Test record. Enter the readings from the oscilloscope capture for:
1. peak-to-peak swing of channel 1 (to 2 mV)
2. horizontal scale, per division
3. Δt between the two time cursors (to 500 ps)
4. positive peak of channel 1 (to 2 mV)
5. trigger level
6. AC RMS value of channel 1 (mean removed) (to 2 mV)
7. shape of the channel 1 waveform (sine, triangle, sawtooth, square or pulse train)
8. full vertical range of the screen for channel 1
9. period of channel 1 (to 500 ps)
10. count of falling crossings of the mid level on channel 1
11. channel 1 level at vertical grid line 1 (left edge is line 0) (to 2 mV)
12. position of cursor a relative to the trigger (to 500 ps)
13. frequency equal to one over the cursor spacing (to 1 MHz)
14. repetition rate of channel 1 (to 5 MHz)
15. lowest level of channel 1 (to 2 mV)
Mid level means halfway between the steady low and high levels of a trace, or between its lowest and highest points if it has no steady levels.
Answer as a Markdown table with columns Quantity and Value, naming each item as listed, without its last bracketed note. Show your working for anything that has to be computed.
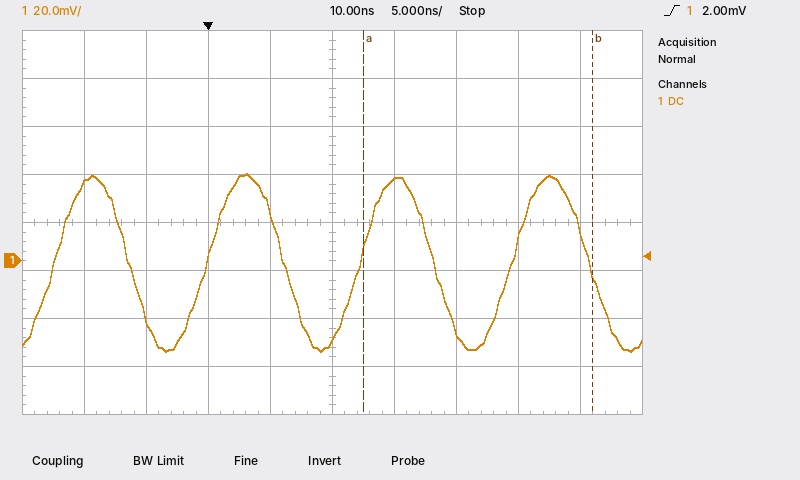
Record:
| Quantity | Value |
|---|---|
| peak-to-peak swing of channel 1 | 36 mV − (-38 mV) = 74 mV |
| horizontal scale, per division | 5 ns |
| Δt between the two time cursors | 18.5 ns |
| positive peak of channel 1 | 36 mV |
| trigger level | 2.00 mV |
| AC RMS value of channel 1 (mean removed) | 74 mV / (2√2) ≈ 26 mV |
| shape of the channel 1 waveform | sine |
| full vertical range of the screen for channel 1 | 160 mV |
| period of channel 1 | 12.5 ns |
| count of falling crossings of the mid level on channel 1 | 4 |
| channel 1 level at vertical grid line 1 (left edge is line 0) | 32 mV |
| position of cursor a relative to the trigger | +12.5 ns |
| frequency equal to one over the cursor spacing | 1 / 18.5 ns ≈ 54 MHz |
| repetition rate of channel 1 | 1 / 12.5 ns ≈ 80 MHz |
| lowest level of channel 1 | -38 mV |
